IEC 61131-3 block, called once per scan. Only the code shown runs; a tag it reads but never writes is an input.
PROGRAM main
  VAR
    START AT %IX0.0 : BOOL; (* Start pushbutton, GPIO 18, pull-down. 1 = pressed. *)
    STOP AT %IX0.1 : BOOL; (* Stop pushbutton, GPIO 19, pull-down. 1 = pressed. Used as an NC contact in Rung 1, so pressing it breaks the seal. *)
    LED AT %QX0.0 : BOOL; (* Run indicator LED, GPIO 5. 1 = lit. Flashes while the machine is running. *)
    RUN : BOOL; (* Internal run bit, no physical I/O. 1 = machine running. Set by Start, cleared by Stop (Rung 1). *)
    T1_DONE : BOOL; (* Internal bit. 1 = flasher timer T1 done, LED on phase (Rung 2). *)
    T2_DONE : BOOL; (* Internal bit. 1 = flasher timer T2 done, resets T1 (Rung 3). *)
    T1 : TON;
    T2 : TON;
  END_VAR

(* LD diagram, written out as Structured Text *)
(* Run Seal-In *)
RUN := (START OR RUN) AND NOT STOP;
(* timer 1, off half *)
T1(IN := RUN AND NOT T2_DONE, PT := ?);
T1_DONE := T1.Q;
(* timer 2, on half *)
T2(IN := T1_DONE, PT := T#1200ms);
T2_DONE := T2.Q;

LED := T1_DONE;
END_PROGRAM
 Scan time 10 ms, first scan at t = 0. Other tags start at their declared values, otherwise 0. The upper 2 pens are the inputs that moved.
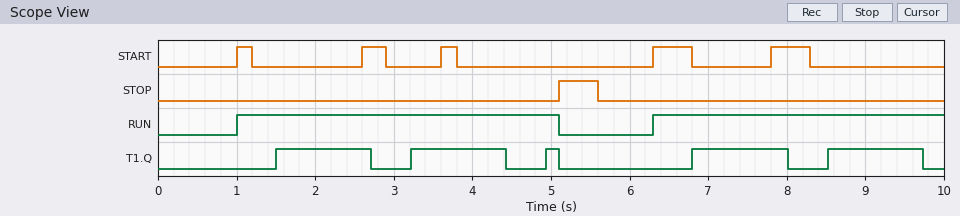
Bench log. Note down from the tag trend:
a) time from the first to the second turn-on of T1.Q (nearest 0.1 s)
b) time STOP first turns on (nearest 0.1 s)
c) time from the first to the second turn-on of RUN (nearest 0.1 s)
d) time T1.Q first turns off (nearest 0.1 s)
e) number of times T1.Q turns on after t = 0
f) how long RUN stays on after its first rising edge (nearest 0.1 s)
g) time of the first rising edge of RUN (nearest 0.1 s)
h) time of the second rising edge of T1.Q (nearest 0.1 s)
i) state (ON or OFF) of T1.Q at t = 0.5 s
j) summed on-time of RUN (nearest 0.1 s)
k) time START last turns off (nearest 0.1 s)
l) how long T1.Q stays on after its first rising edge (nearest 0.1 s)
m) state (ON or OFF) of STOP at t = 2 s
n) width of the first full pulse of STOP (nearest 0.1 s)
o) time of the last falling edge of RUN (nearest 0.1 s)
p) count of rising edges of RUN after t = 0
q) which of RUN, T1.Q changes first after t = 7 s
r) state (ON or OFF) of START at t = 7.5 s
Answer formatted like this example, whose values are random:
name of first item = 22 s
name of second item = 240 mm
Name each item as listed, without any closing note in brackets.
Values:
time from the first to the second turn-on of T1.Q = 1.7 s
time STOP first turns on = 5.1 s
time from the first to the second turn-on of RUN = 5.3 s
time T1.Q first turns off = 2.7 s
number of times T1.Q turns on after t = 0 = 5
how long RUN stays on after its first rising edge = 4.1 s
time of the first rising edge of RUN = 1.0 s
time of the second rising edge of T1.Q = 3.2 s
state (ON or OFF) of T1.Q at t = 0.5 s = OFF
summed on-time of RUN = 7.8 s
time START last turns off = 8.3 s
how long T1.Q stays on after its first rising edge = 1.2 s
state (ON or OFF) of STOP at t = 2 s = OFF
width of the first full pulse of STOP = 0.5 s
time of the last falling edge of RUN = 5.1 s
count of rising edges of RUN after t = 0 = 2
which of RUN, T1.Q changes first after t = 7 s = T1.Q
state (ON or OFF) of START at t = 7.5 s = OFF
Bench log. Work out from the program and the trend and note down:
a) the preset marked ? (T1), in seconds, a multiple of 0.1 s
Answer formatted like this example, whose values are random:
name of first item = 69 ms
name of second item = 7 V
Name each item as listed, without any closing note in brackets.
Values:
the preset marked ? (T1), in seconds, a multiple of 0.1 s = 0.5 s
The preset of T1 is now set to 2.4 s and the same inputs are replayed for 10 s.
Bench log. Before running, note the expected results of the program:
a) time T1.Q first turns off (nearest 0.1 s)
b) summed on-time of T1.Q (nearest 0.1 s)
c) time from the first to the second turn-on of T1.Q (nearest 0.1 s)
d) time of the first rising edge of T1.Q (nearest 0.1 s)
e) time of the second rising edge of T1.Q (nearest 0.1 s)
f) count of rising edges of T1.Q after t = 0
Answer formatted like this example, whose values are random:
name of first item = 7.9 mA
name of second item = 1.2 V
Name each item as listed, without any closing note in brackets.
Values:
time T1.Q first turns off = 4.6 s
summed on-time of T1.Q = 2.4 s
time from the first to the second turn-on of T1.Q = 5.3 s
time of the first rising edge of T1.Q = 3.4 s
time of the second rising edge of T1.Q = 8.7 s
count of rising edges of T1.Q after t = 0 = 2
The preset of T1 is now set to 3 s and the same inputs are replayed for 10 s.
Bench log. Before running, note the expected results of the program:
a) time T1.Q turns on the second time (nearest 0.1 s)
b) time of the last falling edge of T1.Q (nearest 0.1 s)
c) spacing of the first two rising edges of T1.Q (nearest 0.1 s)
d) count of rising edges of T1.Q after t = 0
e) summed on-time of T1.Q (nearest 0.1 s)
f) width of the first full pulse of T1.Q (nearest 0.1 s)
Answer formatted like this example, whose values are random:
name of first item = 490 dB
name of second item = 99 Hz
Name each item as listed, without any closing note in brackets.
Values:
time T1.Q turns on the second time = 9.3 s
time of the last falling edge of T1.Q = 5.1 s
spacing of the first two rising edges of T1.Q = 5.3 s
count of rising edges of T1.Q after t = 0 = 2
summed on-time of T1.Q = 1.8 s
width of the first full pulse of T1.Q = 1.1 s
